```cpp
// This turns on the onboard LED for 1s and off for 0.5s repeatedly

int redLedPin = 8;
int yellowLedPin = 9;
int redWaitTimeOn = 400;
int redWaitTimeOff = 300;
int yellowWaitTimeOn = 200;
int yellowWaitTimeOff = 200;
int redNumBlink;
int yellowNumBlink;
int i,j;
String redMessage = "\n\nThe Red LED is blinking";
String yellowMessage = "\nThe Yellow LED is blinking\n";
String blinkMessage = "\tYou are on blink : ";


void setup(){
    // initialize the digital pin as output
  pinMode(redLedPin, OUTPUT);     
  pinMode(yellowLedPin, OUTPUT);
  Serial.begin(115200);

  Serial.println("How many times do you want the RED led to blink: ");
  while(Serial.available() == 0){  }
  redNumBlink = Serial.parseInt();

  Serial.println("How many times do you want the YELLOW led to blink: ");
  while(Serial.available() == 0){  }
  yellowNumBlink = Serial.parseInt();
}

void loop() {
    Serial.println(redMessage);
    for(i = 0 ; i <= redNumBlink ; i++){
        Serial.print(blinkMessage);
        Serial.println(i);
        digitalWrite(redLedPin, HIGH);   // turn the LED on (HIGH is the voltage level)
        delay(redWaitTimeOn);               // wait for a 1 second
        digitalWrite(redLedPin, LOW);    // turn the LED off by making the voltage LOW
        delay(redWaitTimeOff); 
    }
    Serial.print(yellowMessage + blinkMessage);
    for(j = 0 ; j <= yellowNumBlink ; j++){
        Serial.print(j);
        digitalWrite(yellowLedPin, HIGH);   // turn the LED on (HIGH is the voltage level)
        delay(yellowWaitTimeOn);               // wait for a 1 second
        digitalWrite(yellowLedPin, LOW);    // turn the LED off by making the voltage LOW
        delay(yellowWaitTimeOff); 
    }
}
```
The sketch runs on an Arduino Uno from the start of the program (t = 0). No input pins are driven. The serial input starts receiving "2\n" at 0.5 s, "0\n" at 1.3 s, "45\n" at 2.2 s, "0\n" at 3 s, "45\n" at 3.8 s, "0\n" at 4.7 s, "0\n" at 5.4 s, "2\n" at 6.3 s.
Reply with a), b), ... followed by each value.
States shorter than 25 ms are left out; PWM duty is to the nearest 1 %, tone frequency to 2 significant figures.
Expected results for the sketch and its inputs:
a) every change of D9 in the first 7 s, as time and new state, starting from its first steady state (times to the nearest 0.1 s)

a) 0 s low; 3.4 s high; 3.6 s low; 5.9 s high; 6.1 s low
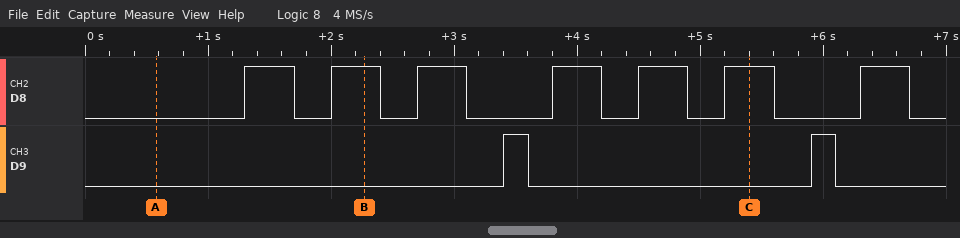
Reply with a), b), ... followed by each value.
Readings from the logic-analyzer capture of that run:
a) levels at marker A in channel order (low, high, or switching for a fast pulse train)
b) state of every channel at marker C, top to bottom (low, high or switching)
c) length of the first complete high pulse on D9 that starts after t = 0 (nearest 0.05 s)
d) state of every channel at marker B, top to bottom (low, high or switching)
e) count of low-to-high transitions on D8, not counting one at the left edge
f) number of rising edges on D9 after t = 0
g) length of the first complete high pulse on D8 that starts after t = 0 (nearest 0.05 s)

a) D8 low, D9 low
b) D8 high, D9 low
c) 0.20 s
d) D8 high, D9 low
e) 7
f) 2
g) 0.40 s
